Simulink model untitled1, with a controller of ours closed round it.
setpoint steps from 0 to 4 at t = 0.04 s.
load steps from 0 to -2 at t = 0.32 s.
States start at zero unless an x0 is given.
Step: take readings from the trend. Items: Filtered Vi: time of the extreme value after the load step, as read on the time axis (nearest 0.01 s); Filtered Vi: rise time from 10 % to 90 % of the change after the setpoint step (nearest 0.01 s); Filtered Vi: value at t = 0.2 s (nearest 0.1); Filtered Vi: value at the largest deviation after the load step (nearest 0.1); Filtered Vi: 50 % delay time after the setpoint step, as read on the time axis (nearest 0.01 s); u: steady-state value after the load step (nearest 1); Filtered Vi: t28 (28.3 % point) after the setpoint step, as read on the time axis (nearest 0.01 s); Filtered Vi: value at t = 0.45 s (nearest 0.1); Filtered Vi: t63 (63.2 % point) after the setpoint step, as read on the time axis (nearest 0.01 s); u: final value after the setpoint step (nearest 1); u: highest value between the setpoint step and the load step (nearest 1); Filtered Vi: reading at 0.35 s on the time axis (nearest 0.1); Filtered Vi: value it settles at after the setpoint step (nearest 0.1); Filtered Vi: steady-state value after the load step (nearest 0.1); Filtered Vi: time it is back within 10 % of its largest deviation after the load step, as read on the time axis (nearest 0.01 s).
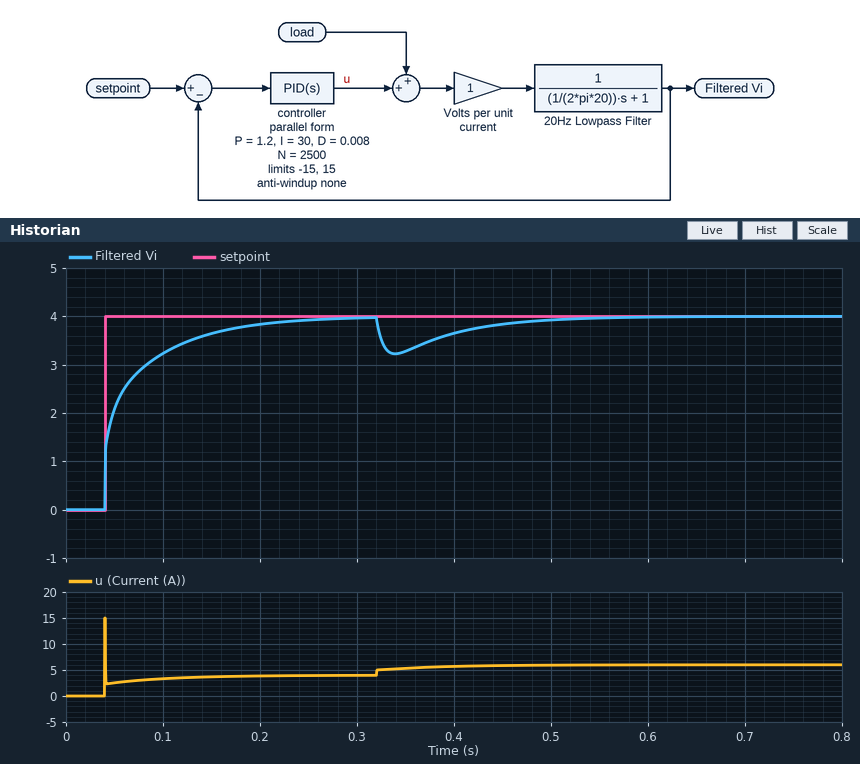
0.34 s
0.10 s
3.8
3.2
0.05 s
6
0.04 s
3.8
0.06 s
4
15
3.3
4.0
4.0
0.50 s
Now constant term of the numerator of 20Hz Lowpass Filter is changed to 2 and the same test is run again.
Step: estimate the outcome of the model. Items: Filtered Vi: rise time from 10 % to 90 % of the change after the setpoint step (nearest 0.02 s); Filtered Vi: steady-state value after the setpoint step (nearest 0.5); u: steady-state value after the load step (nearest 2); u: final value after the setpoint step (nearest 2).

0.06 s
4.0
4
2
